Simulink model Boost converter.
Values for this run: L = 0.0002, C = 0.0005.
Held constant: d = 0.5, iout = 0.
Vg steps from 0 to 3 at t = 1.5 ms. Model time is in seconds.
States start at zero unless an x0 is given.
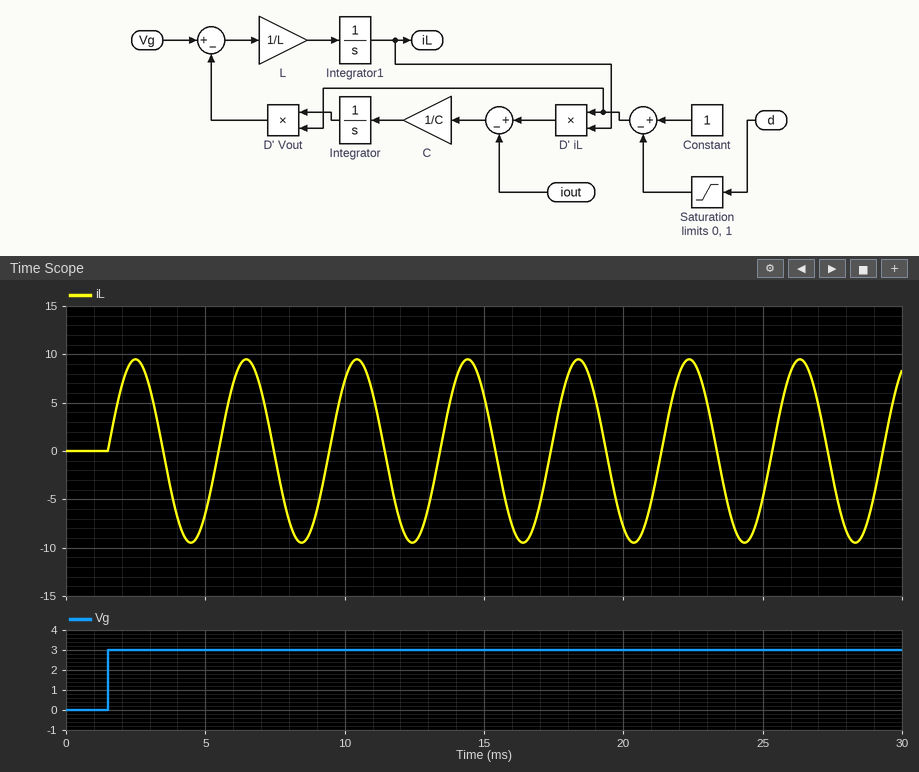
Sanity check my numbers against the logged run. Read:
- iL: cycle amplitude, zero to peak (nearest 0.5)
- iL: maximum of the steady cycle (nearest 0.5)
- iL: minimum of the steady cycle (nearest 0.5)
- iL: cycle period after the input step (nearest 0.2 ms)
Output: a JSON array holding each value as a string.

["9.5", "9.5", "-9.5", "4.0 ms"]
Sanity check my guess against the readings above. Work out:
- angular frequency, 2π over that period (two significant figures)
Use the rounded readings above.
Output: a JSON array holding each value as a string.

["1.6 rad/ms"]
